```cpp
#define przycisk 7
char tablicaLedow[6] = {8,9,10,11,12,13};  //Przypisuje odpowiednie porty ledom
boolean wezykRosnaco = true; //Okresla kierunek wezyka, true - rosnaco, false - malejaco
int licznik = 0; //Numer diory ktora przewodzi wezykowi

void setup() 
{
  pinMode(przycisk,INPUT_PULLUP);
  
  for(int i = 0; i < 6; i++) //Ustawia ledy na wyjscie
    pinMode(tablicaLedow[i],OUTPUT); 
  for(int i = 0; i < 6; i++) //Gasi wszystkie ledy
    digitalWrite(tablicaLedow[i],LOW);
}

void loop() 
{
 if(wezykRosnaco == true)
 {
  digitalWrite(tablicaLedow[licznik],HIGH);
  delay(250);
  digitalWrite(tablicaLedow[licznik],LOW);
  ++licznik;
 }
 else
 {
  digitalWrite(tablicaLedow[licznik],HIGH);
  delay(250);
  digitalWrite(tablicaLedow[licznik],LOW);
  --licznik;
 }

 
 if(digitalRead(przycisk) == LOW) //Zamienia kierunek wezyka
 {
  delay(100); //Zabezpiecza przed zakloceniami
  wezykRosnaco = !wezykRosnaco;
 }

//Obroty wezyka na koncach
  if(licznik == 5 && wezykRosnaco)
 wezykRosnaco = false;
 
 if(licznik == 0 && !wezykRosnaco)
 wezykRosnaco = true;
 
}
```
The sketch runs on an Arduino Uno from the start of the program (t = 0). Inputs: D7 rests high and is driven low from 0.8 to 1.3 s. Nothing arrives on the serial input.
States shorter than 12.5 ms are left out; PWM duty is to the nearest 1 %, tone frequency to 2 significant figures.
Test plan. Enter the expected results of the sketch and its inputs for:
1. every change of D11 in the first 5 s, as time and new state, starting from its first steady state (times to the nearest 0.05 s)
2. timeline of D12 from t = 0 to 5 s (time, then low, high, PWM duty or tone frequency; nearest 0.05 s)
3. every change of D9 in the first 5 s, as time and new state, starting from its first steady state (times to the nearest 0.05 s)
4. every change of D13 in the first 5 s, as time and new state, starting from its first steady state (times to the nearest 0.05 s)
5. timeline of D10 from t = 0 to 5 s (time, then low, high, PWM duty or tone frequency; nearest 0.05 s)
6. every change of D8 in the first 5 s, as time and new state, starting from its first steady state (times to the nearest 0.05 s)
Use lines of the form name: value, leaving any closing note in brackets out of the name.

every change of D11 in the first 5 s, as time and new state, starting from its first steady state: 0 s low; 0.75 s high; 1 s low; 1.35 s high; 1.6 s low; 2.85 s high; 3.1 s low; 3.85 s high; 4.1 s low
timeline of D12 from t = 0 to 5 s: 0 s low; 1.1 s high; 1.35 s low; 3.1 s high; 3.35 s low; 3.6 s high; 3.85 s low
every change of D9 in the first 5 s, as time and new state, starting from its first steady state: 0 s low; 0.25 s high; 0.5 s low; 1.85 s high; 2.1 s low; 2.35 s high; 2.6 s low; 4.35 s high; 4.6 s low; 4.85 s high
every change of D13 in the first 5 s, as time and new state, starting from its first steady state: 0 s low; 3.35 s high; 3.6 s low
timeline of D10 from t = 0 to 5 s: 0 s low; 0.5 s high; 0.75 s low; 1.6 s high; 1.85 s low; 2.6 s high; 2.85 s low; 4.1 s high; 4.35 s low
every change of D8 in the first 5 s, as time and new state, starting from its first steady state: 0 s high; 0.25 s low; 2.1 s high; 2.35 s low; 4.6 s high; 4.85 s low
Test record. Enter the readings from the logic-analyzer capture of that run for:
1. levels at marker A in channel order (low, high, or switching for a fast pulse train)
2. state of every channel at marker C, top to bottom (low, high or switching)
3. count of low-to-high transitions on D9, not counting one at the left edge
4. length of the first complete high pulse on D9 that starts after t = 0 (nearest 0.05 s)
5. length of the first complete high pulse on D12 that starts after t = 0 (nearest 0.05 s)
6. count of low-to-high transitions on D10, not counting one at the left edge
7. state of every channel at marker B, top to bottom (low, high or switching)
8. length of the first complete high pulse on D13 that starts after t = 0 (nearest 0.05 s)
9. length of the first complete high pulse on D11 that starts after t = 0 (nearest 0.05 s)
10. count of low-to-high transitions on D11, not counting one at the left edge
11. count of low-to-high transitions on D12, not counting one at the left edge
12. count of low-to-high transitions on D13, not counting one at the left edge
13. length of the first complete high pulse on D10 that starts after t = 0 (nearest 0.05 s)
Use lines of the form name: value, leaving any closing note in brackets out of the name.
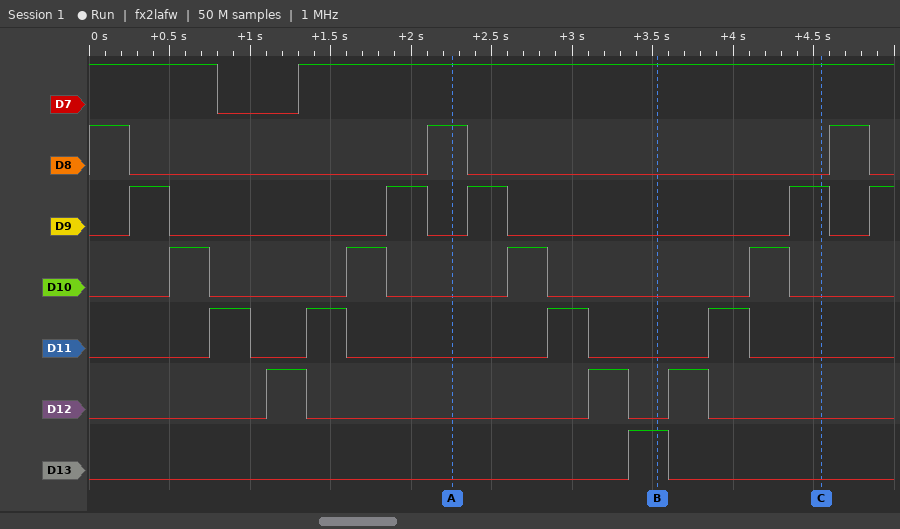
levels at marker A in channel order: D7 high, D8 high, D9 low, D10 low, D11 low, D12 low, D13 low
state of every channel at marker C, top to bottom: D7 high, D8 low, D9 high, D10 low, D11 low, D12 low, D13 low
count of low-to-high transitions on D9, not counting one at the left edge: 5
length of the first complete high pulse on D9 that starts after t = 0: 0.25 s
length of the first complete high pulse on D12 that starts after t = 0: 0.25 s
count of low-to-high transitions on D10, not counting one at the left edge: 4
state of every channel at marker B, top to bottom: D7 high, D8 low, D9 low, D10 low, D11 low, D12 low, D13 high
length of the first complete high pulse on D13 that starts after t = 0: 0.25 s
length of the first complete high pulse on D11 that starts after t = 0: 0.25 s
count of low-to-high transitions on D11, not counting one at the left edge: 4
count of low-to-high transitions on D12, not counting one at the left edge: 3
count of low-to-high transitions on D13, not counting one at the left edge: 1
length of the first complete high pulse on D10 that starts after t = 0: 0.25 s
